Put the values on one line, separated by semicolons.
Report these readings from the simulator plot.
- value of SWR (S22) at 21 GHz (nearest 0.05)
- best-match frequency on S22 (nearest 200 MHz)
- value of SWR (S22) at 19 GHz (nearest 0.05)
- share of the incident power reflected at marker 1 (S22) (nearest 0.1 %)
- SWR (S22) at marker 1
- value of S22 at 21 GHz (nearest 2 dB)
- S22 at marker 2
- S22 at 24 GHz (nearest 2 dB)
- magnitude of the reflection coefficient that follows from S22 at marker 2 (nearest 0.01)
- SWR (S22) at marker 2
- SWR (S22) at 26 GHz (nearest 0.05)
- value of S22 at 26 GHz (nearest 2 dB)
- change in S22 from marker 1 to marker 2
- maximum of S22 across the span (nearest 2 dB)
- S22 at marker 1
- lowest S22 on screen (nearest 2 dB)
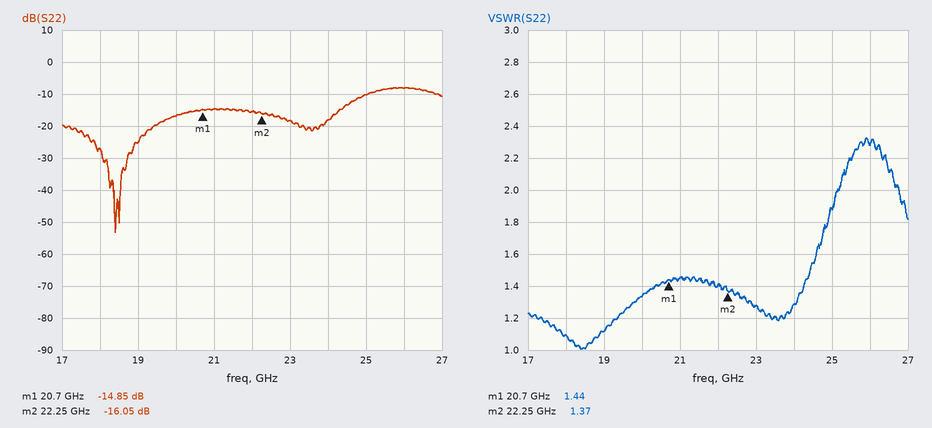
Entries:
1.45; 18.4 GHz; 1.10; 3.3 %; 1.44; -14 dB; -16.05 dB; -18 dB; 0.16; 1.37; 2.30; -8 dB; -1.20 dB; -8 dB; -14.85 dB; -54 dB
